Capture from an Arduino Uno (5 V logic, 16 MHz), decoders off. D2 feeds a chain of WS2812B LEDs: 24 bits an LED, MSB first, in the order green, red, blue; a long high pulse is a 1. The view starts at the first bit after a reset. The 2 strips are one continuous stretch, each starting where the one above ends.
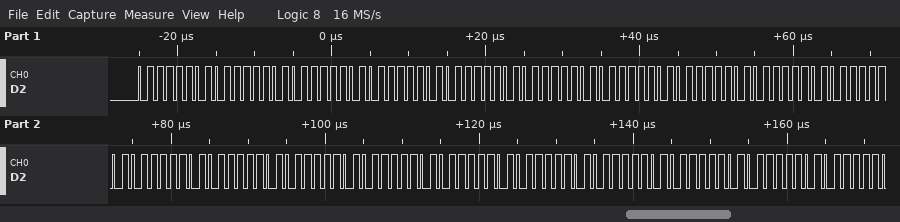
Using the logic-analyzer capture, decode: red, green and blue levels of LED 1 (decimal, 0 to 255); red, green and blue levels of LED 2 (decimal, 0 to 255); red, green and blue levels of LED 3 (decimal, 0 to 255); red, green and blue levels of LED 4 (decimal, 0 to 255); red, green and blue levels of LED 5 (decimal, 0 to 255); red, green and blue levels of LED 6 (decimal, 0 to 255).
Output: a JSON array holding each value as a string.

["125, 125, 125", "125, 125, 125", "125, 125, 125", "125, 125, 125", "125, 125, 125", "125, 125, 125"]
